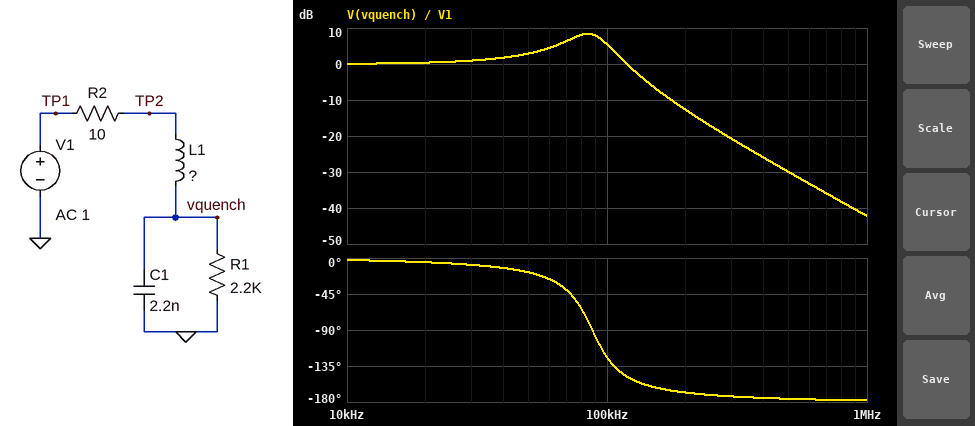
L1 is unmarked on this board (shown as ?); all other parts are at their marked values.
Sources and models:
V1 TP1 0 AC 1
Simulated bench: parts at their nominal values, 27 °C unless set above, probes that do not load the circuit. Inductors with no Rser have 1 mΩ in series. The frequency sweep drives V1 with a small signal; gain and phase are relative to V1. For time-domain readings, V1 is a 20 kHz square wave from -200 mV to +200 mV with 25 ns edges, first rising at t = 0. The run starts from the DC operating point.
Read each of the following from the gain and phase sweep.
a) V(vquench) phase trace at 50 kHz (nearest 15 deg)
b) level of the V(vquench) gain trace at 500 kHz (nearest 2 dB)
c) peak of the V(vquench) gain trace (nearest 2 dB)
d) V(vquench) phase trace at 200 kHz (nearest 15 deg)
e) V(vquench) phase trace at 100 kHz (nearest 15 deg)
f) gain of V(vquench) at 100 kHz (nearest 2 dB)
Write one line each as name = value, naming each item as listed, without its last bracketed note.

V(vquench) phase trace at 50 kHz = -15 deg
level of the V(vquench) gain trace at 500 kHz = -30 dB
peak of the V(vquench) gain trace = 8 dB
V(vquench) phase trace at 200 kHz = -165 deg
V(vquench) phase trace at 100 kHz = -120 deg
gain of V(vquench) at 100 kHz = 6 dB
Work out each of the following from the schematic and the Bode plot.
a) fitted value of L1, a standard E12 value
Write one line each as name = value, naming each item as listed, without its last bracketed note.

fitted value of L1, a standard E12 value = 1.5 mH
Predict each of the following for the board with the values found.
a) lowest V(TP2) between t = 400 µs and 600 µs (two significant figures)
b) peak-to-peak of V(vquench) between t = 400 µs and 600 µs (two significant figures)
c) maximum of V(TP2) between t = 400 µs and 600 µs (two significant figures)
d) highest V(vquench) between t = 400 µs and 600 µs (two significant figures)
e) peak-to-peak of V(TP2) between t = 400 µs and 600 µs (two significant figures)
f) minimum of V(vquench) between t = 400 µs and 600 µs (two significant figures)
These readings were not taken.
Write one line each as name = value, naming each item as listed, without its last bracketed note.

lowest V(TP2) between t = 400 µs and 600 µs = -200 mV
peak-to-peak of V(vquench) between t = 400 µs and 600 µs = 810 mV
maximum of V(TP2) between t = 400 µs and 600 µs = 200 mV
highest V(vquench) between t = 400 µs and 600 µs = 400 mV
peak-to-peak of V(TP2) between t = 400 µs and 600 µs = 400 mV
minimum of V(vquench) between t = 400 µs and 600 µs = -400 mV
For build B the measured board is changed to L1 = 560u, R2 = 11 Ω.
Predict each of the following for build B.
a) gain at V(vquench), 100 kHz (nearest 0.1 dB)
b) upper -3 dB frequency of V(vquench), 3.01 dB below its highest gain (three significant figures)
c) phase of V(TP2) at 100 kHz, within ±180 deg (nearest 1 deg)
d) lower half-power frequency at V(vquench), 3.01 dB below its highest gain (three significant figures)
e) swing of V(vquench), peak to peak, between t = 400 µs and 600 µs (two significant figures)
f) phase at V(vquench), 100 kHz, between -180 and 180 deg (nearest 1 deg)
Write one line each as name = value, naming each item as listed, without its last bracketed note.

gain at V(vquench), 100 kHz = 5.2 dB
upper -3 dB frequency of V(vquench), 3.01 dB below its highest gain = 159 kHz
phase of V(TP2) at 100 kHz, within ±180 deg = -1 deg
lower half-power frequency at V(vquench), 3.01 dB below its highest gain = 122 kHz
swing of V(vquench), peak to peak, between t = 400 µs and 600 µs = 970 mV
phase at V(vquench), 100 kHz, between -180 and 180 deg = -19 deg
